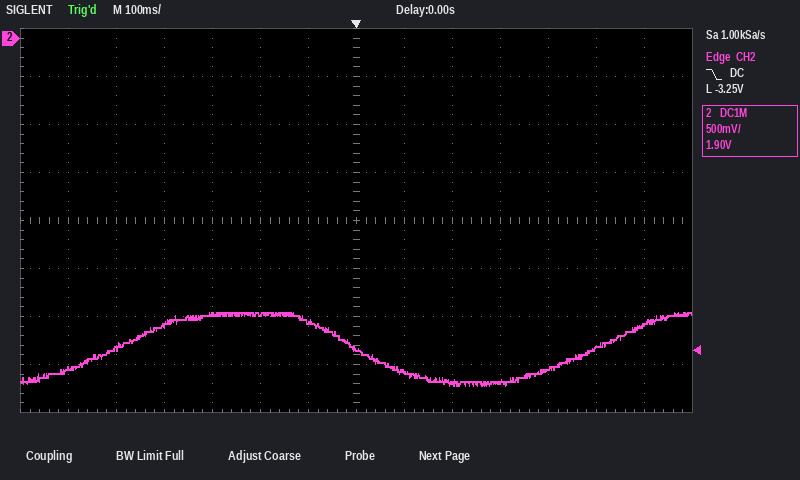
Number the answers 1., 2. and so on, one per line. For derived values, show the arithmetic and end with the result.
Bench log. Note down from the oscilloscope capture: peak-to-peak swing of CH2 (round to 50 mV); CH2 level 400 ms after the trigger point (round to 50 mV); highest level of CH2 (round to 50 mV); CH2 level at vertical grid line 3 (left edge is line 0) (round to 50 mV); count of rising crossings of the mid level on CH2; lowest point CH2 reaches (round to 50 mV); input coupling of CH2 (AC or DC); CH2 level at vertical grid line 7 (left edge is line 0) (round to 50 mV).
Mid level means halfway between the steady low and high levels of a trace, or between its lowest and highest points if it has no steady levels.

1. -2.85 V − (-3.60 V) = 750 mV
2. -3.45 V
3. -2.85 V
4. -3.00 V
5. 2
6. -3.60 V
7. DC
8. -3.25 V
